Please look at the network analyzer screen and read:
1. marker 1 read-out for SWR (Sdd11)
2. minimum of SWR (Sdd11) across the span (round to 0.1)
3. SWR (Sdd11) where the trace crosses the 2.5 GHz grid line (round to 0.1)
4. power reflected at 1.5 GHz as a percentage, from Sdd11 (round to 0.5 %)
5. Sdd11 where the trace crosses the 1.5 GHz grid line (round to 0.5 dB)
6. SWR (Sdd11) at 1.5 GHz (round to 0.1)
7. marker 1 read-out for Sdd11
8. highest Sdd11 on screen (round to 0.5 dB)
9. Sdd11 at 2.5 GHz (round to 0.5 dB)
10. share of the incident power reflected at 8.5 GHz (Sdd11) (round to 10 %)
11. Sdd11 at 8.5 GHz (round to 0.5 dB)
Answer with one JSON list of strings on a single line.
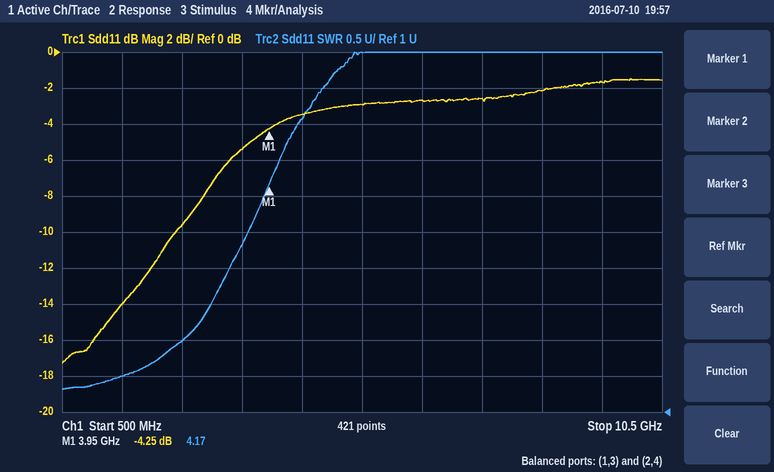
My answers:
["4.17", "1.3", "2.0", "4.0 %", "-14.0 dB", "1.5", "-4.25 dB", "-1.5 dB", "-9.5 dB", "60 %", "-2.0 dB"]
